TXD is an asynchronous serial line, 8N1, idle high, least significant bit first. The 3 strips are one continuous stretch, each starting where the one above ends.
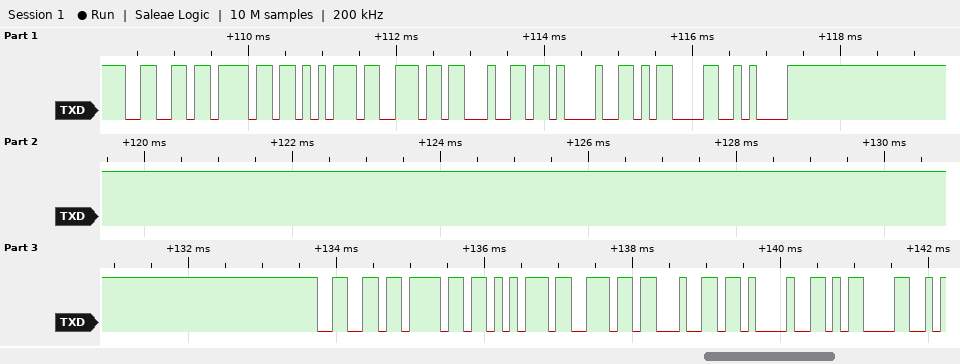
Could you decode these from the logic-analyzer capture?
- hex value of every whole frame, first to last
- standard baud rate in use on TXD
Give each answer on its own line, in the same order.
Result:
66 6F 75 6E 64 21 0D 0A 66 6F 75 6E 64 21 0D
9600 baud
